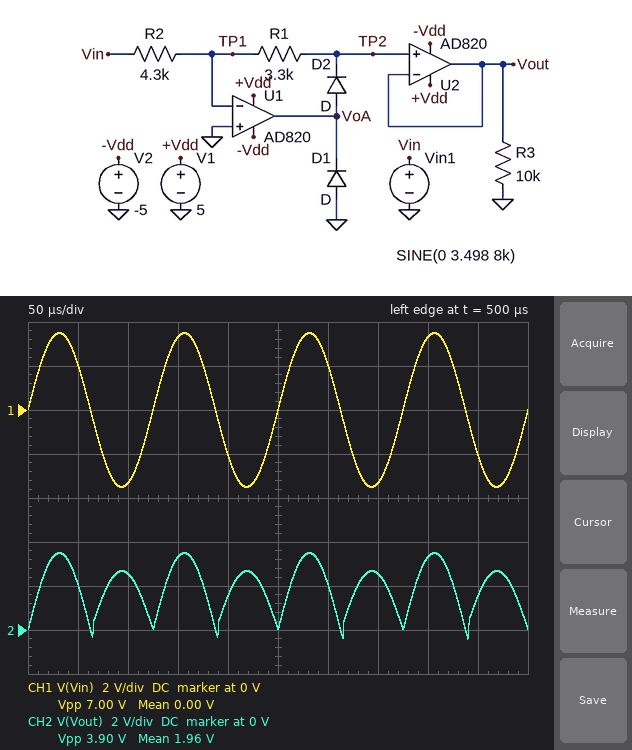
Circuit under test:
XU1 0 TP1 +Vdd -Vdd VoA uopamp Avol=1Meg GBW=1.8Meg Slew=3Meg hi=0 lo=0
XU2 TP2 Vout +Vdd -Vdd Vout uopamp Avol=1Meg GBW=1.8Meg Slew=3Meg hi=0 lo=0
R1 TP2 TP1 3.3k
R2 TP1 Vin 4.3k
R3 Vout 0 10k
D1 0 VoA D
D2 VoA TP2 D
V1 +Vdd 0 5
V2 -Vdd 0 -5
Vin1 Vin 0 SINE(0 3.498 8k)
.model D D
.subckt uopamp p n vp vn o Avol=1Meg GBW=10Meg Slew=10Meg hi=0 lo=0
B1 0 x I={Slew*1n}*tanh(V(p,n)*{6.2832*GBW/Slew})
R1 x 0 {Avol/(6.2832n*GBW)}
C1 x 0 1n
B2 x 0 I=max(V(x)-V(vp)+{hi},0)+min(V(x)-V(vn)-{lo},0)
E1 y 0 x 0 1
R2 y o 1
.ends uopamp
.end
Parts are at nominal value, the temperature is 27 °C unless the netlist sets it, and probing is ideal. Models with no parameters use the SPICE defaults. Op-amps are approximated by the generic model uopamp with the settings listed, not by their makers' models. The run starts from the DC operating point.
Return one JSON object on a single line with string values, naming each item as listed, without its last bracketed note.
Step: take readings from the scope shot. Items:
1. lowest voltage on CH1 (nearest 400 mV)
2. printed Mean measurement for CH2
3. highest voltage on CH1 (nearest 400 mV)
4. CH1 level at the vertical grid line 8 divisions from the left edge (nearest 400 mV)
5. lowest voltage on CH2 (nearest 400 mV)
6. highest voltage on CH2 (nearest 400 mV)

{"lowest voltage on CH1": "-3.6 V", "printed Mean measurement for CH2": "1.96 V", "highest voltage on CH1": "3.6 V", "CH1 level at the vertical grid line 8 divisions from the left edge": "3.2 V", "lowest voltage on CH2": "-400 mV", "highest voltage on CH2": "3.6 V"}
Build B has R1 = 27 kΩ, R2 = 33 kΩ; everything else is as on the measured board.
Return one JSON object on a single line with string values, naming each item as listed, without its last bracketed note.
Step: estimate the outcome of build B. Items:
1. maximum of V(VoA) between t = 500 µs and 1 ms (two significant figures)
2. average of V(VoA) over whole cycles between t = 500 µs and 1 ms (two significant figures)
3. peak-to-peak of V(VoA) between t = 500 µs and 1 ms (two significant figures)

{"maximum of V(VoA) between t = 500 µs and 1 ms": "3.5 V", "average of V(VoA) over whole cycles between t = 500 µs and 1 ms": "740 mV", "peak-to-peak of V(VoA) between t = 500 µs and 1 ms": "4.3 V"}
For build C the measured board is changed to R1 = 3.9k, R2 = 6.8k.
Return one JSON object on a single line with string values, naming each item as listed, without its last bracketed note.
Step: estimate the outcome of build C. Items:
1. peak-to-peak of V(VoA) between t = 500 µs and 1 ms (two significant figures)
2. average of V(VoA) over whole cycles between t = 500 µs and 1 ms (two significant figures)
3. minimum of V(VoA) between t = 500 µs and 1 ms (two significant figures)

{"peak-to-peak of V(VoA) between t = 500 µs and 1 ms": "3.5 V", "average of V(VoA) over whole cycles between t = 500 µs and 1 ms": "490 mV", "minimum of V(VoA) between t = 500 µs and 1 ms": "-870 mV"}
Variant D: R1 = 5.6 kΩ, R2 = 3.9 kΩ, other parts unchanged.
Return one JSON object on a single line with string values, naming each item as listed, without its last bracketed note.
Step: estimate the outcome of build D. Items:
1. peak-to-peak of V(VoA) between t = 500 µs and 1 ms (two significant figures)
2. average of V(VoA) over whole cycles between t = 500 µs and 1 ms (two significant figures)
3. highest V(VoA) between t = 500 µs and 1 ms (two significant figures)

{"peak-to-peak of V(VoA) between t = 500 µs and 1 ms": "5.9 V", "average of V(VoA) over whole cycles between t = 500 µs and 1 ms": "1.4 V", "highest V(VoA) between t = 500 µs and 1 ms": "5.0 V"}
